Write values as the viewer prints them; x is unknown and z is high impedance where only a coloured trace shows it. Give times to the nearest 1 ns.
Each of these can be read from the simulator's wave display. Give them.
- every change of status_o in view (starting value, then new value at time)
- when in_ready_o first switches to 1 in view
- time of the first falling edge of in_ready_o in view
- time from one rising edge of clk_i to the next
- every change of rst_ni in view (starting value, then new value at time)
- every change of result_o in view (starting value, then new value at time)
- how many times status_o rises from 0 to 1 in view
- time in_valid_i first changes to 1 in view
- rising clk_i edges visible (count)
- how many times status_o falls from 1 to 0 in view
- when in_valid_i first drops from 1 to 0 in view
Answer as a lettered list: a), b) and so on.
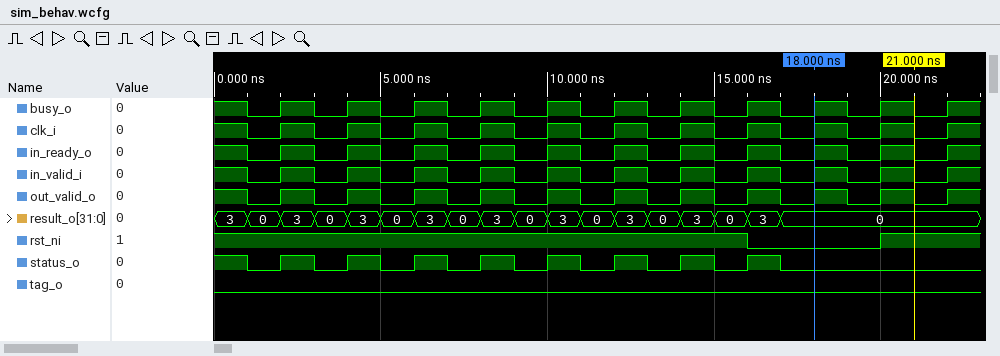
a) 1, 0 at 1 ns, 1 at 2 ns, 0 at 3 ns, 1 at 4 ns, 0 at 5 ns, 1 at 6 ns, 0 at 7 ns, 1 at 8 ns, 0 at 9 ns, 1 at 10 ns, 0 at 11 ns, 1 at 12 ns, 0 at 13 ns, 1 at 14 ns, 0 at 15 ns, 1 at 16 ns, 0 at 17 ns
b) 2 ns
c) 1 ns
d) 2 ns
e) 1, 0 at 16 ns, 1 at 20 ns
f) 3, 0 at 1 ns, 3 at 2 ns, 0 at 3 ns, 3 at 4 ns, 0 at 5 ns, 3 at 6 ns, 0 at 7 ns, 3 at 8 ns, 0 at 9 ns, 3 at 10 ns, 0 at 11 ns, 3 at 12 ns, 0 at 13 ns, 3 at 14 ns, 0 at 15 ns, 3 at 16 ns, 0 at 17 ns
g) 8
h) 2 ns
i) 11
j) 9
k) 1 ns
